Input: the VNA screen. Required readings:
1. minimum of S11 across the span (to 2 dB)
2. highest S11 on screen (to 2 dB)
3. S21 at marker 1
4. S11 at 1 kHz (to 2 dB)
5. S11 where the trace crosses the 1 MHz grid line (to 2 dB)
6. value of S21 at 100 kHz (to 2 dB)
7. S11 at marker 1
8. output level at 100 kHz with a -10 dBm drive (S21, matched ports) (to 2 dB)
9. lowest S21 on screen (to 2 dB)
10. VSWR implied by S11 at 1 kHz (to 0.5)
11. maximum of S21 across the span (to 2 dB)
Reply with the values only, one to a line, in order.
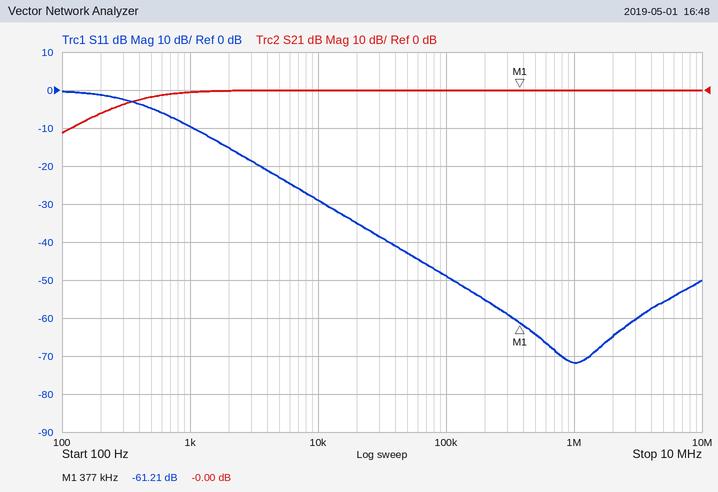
-72 dB
0 dB
-0.00 dB
-10 dB
-72 dB
0 dB
-61.21 dB
-10 dBm
-12 dB
2.0
0 dB
